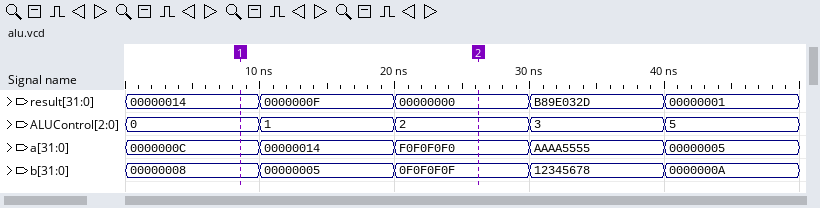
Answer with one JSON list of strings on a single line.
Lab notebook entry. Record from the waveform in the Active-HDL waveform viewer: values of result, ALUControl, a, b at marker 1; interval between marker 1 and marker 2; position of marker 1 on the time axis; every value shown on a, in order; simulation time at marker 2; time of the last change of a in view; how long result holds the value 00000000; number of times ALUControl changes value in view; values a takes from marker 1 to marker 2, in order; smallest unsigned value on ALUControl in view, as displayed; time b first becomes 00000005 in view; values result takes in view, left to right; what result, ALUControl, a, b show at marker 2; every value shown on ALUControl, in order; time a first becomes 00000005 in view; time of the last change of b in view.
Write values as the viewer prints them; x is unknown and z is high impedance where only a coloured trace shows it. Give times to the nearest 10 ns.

["result=00000014, ALUControl=0, a=0000000C, b=00000008", "20 ns", "10 ns", "0000000C, 00000014, F0F0F0F0, AAAA5555, 00000005", "30 ns", "40 ns", "10 ns", "4", "0000000C, 00000014, F0F0F0F0", "0", "10 ns", "00000014, 0000000F, 00000000, B89E032D, 00000001", "result=00000000, ALUControl=2, a=F0F0F0F0, b=0F0F0F0F", "0, 1, 2, 3, 5", "40 ns", "40 ns"]
